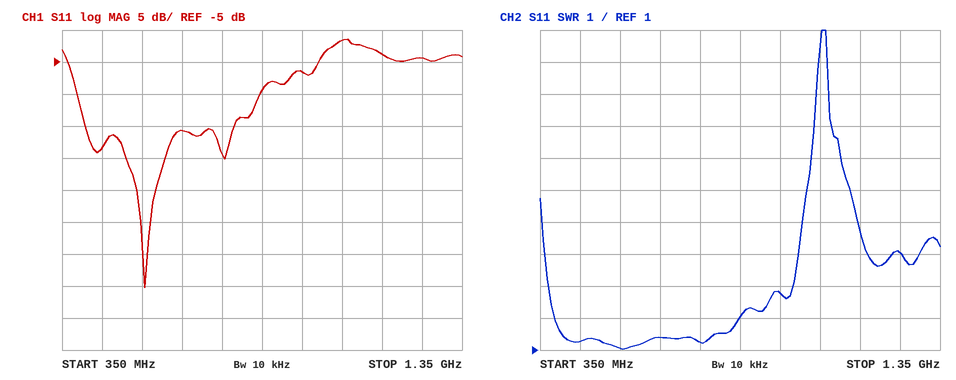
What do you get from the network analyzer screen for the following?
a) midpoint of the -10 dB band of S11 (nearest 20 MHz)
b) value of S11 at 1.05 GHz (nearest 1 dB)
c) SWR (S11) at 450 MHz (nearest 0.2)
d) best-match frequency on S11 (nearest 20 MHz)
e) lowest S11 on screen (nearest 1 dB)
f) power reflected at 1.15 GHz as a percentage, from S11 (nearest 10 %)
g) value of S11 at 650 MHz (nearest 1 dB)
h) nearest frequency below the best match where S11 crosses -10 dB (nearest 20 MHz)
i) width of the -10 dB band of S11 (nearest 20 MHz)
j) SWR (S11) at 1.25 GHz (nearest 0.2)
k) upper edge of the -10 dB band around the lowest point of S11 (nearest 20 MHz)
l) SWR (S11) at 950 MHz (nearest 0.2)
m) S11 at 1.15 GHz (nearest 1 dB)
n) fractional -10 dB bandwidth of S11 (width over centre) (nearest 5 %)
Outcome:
620 MHz
-2 dB
1.2
560 MHz
-40 dB
40 %
-16 dB
380 MHz
460 MHz
4.0
840 MHz
2.8
-4 dB
75 %
